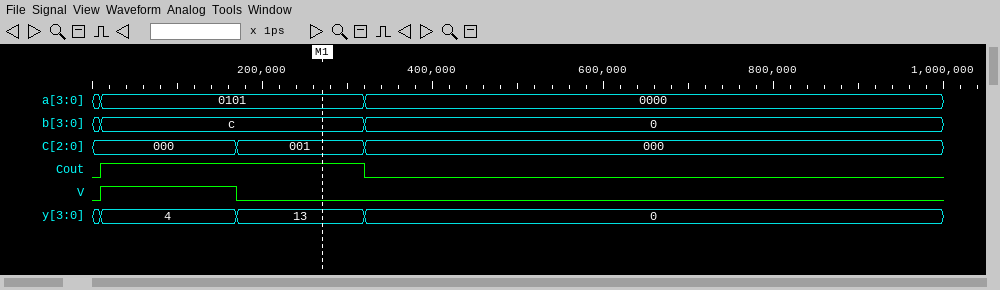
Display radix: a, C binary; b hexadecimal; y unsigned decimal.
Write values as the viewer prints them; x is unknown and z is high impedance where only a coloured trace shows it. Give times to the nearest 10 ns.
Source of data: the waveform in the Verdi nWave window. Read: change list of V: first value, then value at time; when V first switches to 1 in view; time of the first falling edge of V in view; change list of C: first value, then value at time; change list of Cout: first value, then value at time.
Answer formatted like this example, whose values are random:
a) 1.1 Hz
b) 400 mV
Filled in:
a) 0, 1 at 10 ns, 0 at 170 ns
b) 10 ns
c) 170 ns
d) 000, 001 at 170 ns, 000 at 320 ns
e) 0, 1 at 10 ns, 0 at 320 ns
